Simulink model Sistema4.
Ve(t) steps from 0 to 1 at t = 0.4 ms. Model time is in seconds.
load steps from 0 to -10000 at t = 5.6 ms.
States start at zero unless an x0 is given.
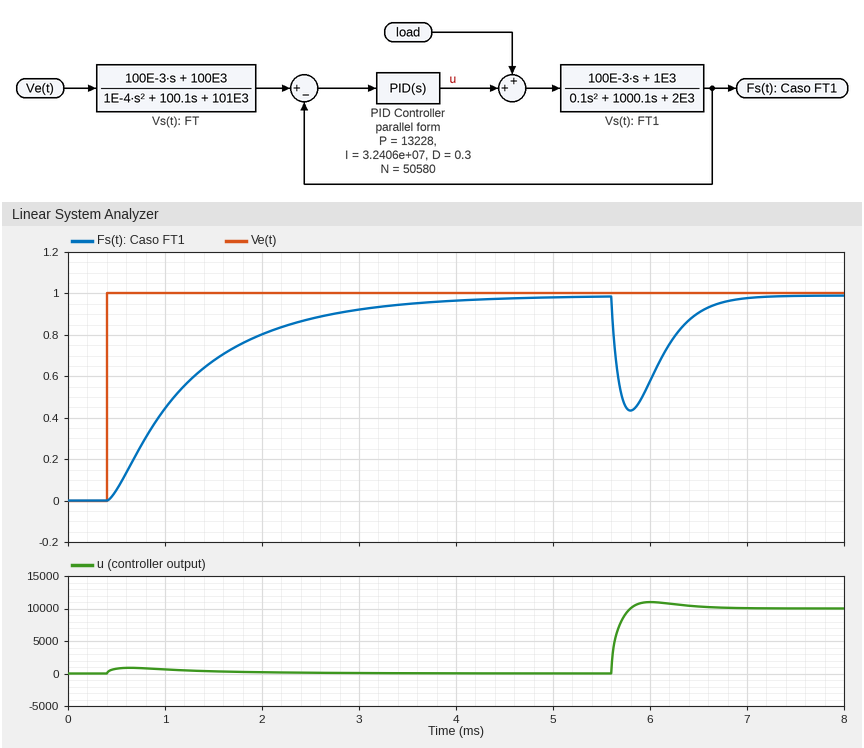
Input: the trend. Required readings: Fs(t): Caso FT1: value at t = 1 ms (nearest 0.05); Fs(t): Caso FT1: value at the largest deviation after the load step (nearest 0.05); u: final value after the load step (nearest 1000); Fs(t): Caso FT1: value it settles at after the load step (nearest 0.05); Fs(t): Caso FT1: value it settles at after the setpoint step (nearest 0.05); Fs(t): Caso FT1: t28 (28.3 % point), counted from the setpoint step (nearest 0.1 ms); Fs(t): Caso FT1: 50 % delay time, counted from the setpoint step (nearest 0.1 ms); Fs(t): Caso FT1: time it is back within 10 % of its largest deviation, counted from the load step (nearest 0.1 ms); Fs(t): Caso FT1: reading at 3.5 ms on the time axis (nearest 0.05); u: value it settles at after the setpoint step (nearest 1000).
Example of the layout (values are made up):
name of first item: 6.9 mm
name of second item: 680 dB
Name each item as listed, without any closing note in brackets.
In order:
Fs(t): Caso FT1: value at t = 1 ms: 0.45
Fs(t): Caso FT1: value at the largest deviation after the load step: 0.45
u: final value after the load step: 10000
Fs(t): Caso FT1: value it settles at after the load step: 1.00
Fs(t): Caso FT1: value it settles at after the setpoint step: 1.00
Fs(t): Caso FT1: t28 (28.3 % point), counted from the setpoint step: 0.4 ms
Fs(t): Caso FT1: 50 % delay time, counted from the setpoint step: 0.7 ms
Fs(t): Caso FT1: time it is back within 10 % of its largest deviation, counted from the load step: 1.0 ms
Fs(t): Caso FT1: reading at 3.5 ms on the time axis: 0.95
u: value it settles at after the setpoint step: 0
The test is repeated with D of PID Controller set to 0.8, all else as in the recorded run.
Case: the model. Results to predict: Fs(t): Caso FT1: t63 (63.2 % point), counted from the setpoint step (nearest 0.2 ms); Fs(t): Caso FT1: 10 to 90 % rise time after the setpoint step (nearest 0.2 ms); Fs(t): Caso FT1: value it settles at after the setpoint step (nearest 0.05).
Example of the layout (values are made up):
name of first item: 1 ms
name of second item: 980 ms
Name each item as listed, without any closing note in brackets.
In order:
Fs(t): Caso FT1: t63 (63.2 % point), counted from the setpoint step: 1.0 ms
Fs(t): Caso FT1: 10 to 90 % rise time after the setpoint step: 2.0 ms
Fs(t): Caso FT1: value it settles at after the setpoint step: 1.00
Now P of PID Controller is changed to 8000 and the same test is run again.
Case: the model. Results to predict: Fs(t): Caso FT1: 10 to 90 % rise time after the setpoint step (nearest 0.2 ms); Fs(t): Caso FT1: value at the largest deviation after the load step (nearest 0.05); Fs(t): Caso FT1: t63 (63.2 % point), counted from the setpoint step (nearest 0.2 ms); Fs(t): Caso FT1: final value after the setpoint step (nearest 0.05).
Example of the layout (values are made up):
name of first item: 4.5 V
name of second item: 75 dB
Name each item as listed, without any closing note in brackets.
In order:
Fs(t): Caso FT1: 10 to 90 % rise time after the setpoint step: 2.0 ms
Fs(t): Caso FT1: value at the largest deviation after the load step: 0.25
Fs(t): Caso FT1: t63 (63.2 % point), counted from the setpoint step: 1.0 ms
Fs(t): Caso FT1: final value after the setpoint step: 1.00
